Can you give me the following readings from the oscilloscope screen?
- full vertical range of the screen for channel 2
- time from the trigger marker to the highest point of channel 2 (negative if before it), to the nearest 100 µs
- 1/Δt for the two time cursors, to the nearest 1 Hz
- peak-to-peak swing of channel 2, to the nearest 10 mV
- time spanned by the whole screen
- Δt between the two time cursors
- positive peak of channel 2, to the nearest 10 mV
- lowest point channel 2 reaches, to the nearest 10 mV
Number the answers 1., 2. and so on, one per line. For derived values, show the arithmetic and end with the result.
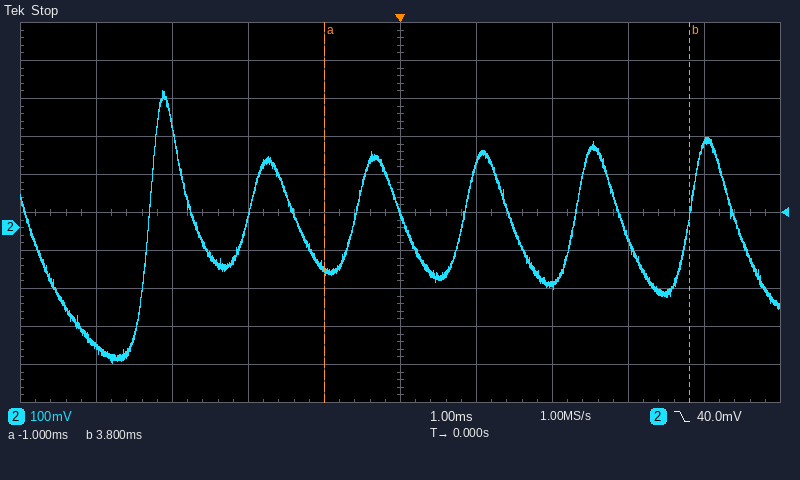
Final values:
1. 1 V
2. -3.1 ms
3. 1 / 4.8 ms ≈ 208 Hz
4. 360 mV − (-360 mV) = 720 mV
5. 10 ms
6. 3.8 ms − (-1 ms) = 4.8 ms
7. 360 mV
8. -360 mV
